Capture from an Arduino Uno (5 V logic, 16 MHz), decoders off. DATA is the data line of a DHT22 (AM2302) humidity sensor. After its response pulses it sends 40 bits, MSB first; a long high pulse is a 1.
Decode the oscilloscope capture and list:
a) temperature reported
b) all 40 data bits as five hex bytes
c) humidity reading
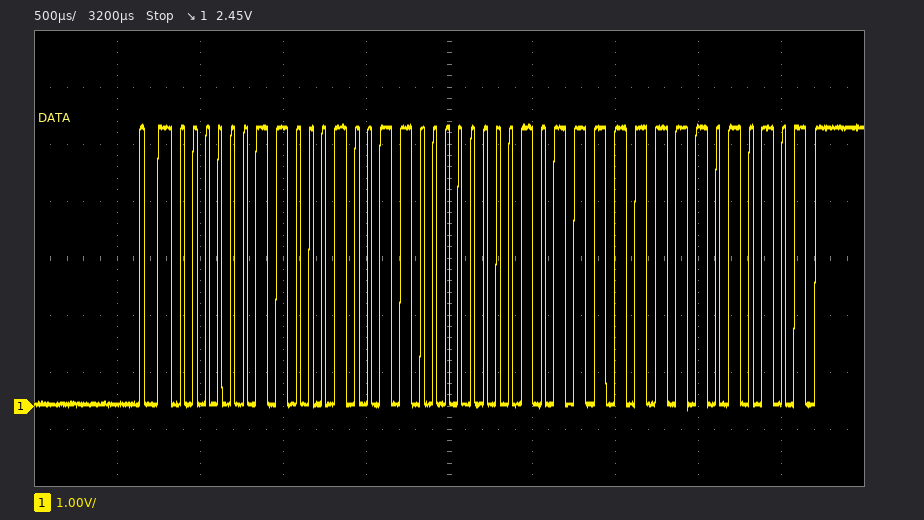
19.1 °C
03 13 00 BF D5
78.7 %
